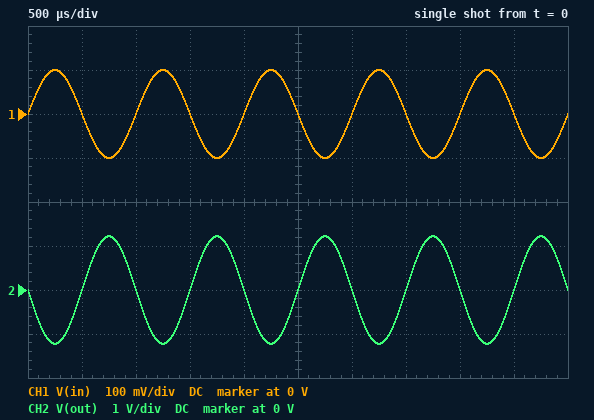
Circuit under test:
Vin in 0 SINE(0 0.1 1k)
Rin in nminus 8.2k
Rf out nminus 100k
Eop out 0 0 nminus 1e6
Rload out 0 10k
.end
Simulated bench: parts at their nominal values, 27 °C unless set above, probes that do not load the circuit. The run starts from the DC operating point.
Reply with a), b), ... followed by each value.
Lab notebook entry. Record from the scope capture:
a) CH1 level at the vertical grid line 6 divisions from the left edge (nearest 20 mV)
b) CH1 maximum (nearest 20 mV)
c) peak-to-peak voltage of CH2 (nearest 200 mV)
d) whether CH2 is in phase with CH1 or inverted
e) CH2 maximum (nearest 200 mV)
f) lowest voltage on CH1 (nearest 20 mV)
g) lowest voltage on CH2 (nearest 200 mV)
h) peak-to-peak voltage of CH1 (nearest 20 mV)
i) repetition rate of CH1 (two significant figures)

a) 0 V
b) 100 mV
c) 2.4 V
d) inverted
e) 1.2 V
f) -100 mV
g) -1.2 V
h) 200 mV
i) 1.0 kHz
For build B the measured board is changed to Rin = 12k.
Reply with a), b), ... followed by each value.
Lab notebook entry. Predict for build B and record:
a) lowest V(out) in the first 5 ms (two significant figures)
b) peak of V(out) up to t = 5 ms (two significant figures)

a) -830 mV
b) 830 mV
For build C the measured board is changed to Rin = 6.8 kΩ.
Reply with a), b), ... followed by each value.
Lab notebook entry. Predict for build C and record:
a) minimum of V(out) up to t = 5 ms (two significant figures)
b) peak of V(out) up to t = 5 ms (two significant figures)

a) -1.5 V
b) 1.5 V
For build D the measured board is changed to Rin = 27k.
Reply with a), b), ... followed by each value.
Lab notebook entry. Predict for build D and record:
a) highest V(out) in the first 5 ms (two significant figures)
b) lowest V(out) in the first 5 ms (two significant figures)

a) 370 mV
b) -370 mV
